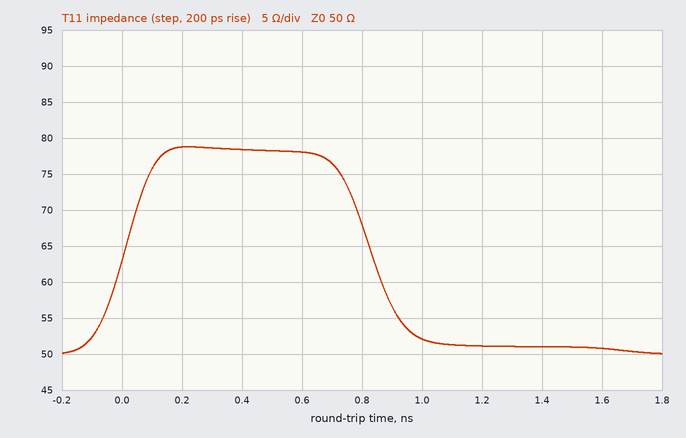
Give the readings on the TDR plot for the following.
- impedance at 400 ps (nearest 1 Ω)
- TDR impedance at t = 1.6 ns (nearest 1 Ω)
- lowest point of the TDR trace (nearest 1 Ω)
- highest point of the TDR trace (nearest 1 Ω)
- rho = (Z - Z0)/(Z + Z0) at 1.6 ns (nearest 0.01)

78 Ω
51 Ω
50 Ω
79 Ω
+0.01
